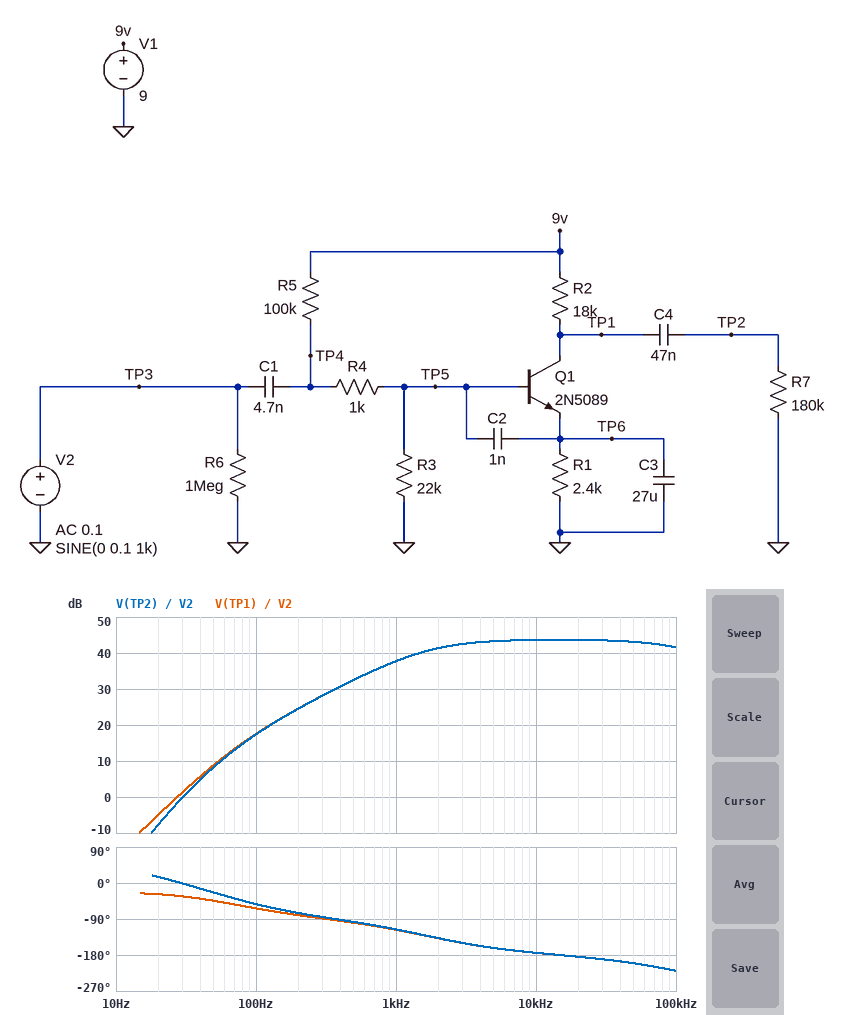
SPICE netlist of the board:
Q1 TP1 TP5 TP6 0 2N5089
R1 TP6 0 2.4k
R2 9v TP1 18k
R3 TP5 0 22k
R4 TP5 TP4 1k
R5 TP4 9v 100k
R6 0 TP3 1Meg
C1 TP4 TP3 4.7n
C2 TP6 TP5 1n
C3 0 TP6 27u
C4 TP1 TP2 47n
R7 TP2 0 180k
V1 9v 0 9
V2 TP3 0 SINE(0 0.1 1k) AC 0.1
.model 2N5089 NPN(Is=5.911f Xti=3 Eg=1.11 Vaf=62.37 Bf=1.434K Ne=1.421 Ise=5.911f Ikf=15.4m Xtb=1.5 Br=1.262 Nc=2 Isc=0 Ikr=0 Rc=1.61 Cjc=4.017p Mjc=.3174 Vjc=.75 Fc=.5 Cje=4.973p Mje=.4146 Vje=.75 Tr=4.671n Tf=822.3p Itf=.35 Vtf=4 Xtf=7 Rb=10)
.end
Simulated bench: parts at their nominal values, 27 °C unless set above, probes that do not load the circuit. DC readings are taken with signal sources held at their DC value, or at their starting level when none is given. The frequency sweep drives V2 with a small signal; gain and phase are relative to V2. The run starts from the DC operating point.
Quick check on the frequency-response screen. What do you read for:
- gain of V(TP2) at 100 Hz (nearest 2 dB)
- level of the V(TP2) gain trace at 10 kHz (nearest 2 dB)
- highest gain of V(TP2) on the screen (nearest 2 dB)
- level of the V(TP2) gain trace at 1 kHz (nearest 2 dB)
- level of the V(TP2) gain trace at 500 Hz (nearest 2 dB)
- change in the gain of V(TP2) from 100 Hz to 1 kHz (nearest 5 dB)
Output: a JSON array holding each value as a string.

["18 dB", "44 dB", "44 dB", "38 dB", "32 dB", "20 dB"]
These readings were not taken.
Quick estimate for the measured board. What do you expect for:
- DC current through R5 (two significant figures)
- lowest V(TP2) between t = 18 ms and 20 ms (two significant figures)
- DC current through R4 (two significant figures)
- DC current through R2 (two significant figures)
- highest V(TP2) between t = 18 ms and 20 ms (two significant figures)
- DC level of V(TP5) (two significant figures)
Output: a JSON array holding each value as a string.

["73 µA", "-1.3 V", "73 µA", "400 µA", "2.7 V", "1.6 V"]
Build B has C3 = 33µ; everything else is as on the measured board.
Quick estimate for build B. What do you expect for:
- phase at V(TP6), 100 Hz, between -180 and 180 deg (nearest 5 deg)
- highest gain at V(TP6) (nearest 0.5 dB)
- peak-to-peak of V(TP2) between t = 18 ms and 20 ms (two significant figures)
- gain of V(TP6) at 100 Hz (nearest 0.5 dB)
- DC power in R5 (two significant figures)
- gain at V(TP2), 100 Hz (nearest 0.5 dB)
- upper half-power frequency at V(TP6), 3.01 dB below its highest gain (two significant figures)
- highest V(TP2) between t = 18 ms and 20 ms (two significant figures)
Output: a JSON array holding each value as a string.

["25 deg", "-32.0 dB", "4.2 V", "-32.5 dB", "540 µW", "18.0 dB", "1.8 kHz", "2.8 V"]
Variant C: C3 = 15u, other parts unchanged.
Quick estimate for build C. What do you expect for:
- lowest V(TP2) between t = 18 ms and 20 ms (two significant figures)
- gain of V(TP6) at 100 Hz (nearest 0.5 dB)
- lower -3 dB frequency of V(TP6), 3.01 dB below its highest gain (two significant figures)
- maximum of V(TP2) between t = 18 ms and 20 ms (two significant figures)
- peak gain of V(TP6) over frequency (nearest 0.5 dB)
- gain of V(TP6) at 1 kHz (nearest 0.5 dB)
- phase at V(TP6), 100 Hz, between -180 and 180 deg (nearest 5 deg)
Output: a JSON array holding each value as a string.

["-1.2 V", "-28.5 dB", "100 Hz", "2.6 V", "-25.5 dB", "-26.0 dB", "45 deg"]
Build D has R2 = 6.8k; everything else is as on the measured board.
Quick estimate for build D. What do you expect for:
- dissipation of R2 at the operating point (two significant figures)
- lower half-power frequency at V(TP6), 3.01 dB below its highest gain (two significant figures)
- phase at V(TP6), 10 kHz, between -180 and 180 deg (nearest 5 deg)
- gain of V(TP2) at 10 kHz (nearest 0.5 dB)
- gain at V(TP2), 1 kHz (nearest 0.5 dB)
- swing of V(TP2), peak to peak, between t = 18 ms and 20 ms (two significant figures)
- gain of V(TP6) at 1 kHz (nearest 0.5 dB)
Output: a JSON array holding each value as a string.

["1.1 mW", "64 Hz", "-80 deg", "37.0 dB", "30.5 dB", "5.9 V", "-30.5 dB"]
